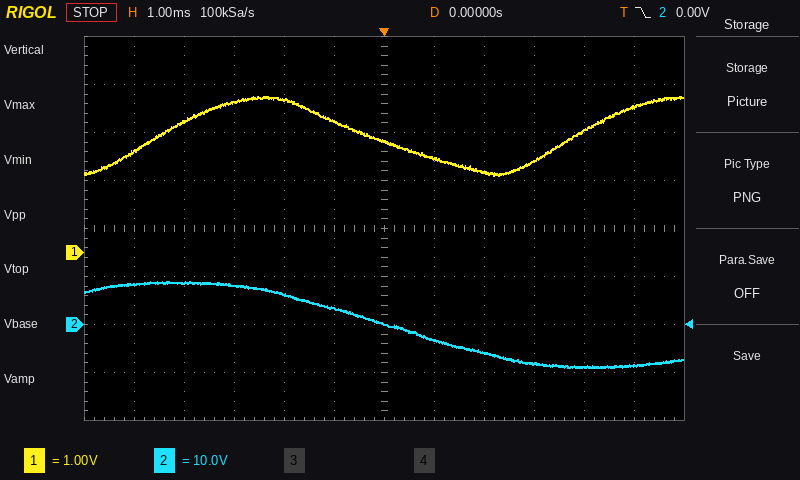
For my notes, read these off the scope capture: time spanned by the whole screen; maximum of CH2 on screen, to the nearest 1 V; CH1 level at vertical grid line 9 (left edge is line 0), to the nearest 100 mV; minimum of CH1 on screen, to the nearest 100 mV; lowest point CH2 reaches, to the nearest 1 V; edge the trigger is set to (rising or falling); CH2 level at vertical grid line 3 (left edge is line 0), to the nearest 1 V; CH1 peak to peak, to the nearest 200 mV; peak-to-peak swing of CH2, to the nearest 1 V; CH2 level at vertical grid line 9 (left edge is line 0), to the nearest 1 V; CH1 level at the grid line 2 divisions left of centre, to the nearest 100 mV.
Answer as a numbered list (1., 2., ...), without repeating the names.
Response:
1. 12 ms
2. 9 V
3. 1.9 V
4. 1.6 V
5. -9 V
6. falling
7. 8 V
8. 1.6 V
9. 18 V
10. -8 V
11. 3.2 V
